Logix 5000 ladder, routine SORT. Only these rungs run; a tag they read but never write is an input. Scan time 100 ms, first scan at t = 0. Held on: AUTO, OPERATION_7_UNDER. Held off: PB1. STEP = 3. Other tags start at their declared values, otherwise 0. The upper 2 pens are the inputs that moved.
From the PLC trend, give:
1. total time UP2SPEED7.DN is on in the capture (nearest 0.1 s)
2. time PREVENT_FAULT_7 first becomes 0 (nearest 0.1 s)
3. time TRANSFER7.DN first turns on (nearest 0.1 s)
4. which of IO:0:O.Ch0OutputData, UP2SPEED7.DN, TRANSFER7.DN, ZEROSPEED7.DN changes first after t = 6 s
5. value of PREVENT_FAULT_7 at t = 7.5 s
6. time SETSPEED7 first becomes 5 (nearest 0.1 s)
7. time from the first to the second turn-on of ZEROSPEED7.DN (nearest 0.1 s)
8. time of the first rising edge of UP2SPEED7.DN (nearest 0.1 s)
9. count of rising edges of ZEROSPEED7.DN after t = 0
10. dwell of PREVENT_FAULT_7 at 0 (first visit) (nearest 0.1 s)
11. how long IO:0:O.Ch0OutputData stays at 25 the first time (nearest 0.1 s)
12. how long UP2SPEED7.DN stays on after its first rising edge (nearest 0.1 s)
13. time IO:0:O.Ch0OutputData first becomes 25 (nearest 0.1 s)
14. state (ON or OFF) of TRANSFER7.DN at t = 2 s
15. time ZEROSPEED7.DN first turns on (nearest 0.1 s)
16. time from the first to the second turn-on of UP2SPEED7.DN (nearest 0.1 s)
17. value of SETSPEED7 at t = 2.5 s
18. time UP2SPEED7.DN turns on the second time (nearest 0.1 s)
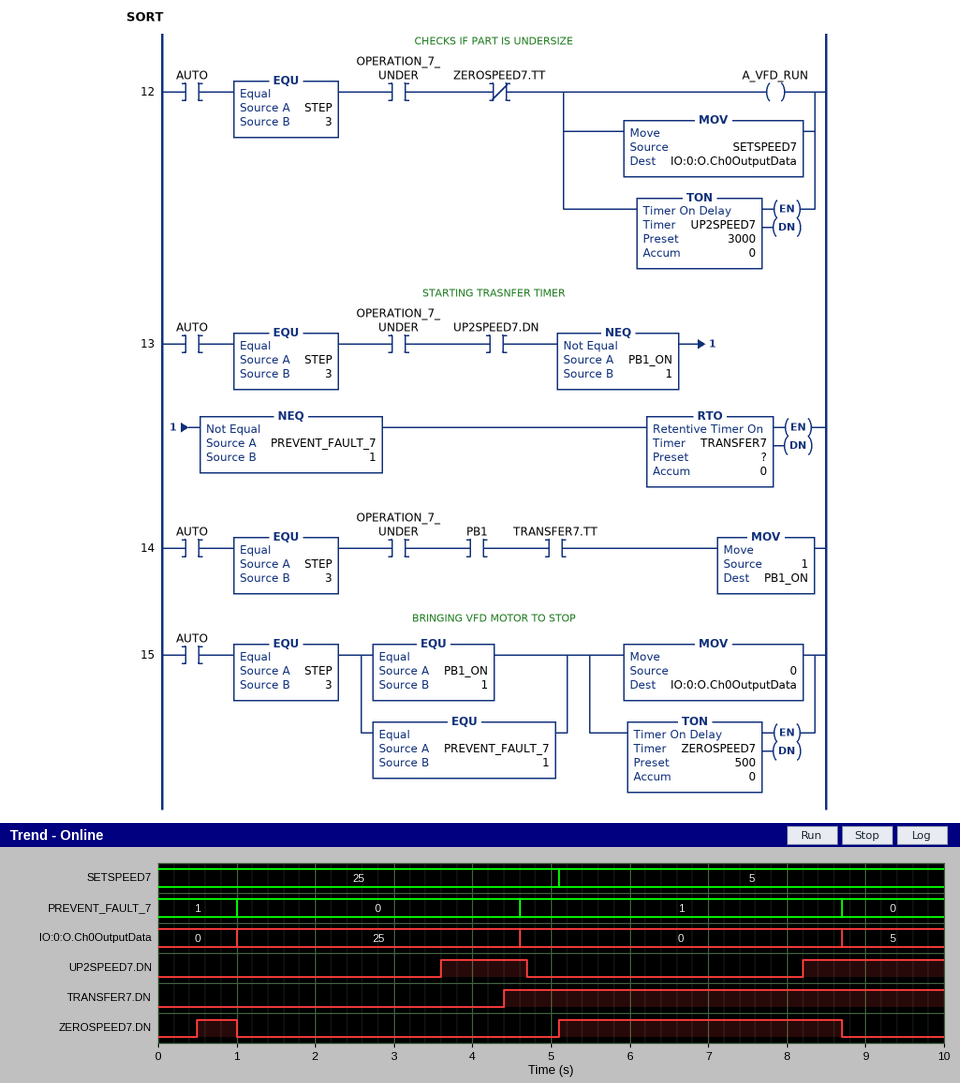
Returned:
2.9 s
1.0 s
4.4 s
UP2SPEED7.DN
1
5.1 s
4.6 s
3.6 s
2
3.6 s
3.6 s
1.1 s
1.0 s
OFF
0.5 s
4.6 s
25
8.2 s
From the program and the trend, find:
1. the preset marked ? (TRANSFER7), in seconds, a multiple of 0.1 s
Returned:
0.8 s
